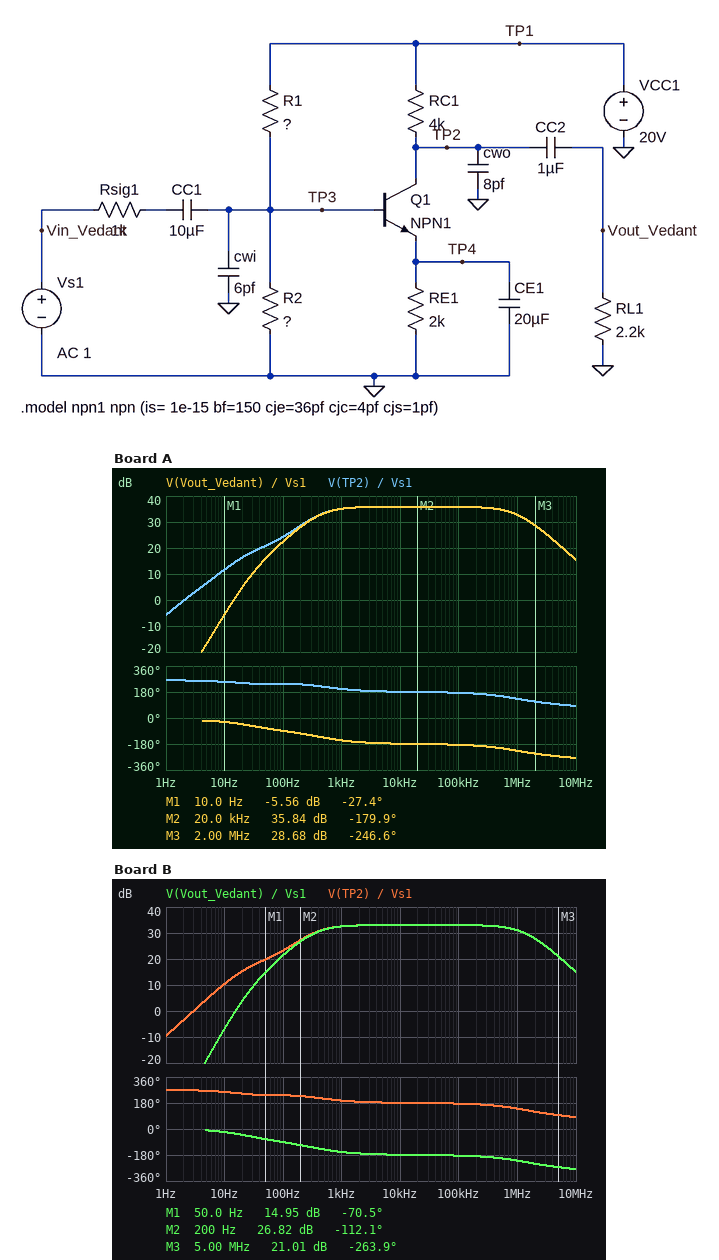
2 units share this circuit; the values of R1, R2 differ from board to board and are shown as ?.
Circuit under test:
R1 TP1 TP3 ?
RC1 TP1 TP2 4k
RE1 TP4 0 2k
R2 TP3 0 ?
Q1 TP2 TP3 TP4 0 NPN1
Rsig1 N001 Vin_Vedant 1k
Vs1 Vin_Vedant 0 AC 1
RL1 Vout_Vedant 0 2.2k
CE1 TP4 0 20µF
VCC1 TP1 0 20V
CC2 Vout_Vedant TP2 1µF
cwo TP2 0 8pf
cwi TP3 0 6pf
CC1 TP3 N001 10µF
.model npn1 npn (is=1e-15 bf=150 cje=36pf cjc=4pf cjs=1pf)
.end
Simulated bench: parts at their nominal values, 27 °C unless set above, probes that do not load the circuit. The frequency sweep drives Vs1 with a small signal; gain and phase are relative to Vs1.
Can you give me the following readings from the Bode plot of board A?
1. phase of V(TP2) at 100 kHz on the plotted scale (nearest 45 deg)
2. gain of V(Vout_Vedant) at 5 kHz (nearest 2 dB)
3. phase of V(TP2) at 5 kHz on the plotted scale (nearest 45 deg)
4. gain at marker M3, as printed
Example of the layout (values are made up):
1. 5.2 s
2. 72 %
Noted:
1. 180 deg
2. 36 dB
3. 180 deg
4. 28.68 dB
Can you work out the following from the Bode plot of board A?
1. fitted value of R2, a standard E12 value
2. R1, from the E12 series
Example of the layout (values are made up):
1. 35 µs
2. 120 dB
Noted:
1. 5.6 kΩ
2. 18 kΩ
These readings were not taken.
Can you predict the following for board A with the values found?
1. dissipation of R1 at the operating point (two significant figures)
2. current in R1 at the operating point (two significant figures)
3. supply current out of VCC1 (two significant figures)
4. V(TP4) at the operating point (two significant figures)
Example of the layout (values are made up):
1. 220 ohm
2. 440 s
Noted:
1. 13 mW
2. 850 µA
3. 2.8 mA
4. 4.0 V
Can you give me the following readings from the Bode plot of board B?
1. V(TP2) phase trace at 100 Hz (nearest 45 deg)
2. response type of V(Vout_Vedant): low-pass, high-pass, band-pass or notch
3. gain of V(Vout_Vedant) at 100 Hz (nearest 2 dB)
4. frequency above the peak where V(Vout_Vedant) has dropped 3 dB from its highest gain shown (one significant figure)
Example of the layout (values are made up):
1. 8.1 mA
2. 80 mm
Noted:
1. 225 deg
2. band-pass
3. 22 dB
4. 1 MHz
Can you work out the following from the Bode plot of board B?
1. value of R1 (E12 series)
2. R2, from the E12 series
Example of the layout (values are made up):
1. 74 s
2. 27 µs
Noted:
1. 15 kΩ
2. 3.3 kΩ
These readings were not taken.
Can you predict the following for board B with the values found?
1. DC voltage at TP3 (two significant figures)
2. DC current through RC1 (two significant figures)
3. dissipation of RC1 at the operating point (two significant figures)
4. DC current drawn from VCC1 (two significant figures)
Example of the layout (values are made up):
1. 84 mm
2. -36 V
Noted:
1. 3.6 V
2. 1.4 mA
3. 8.1 mW
4. 2.5 mA
